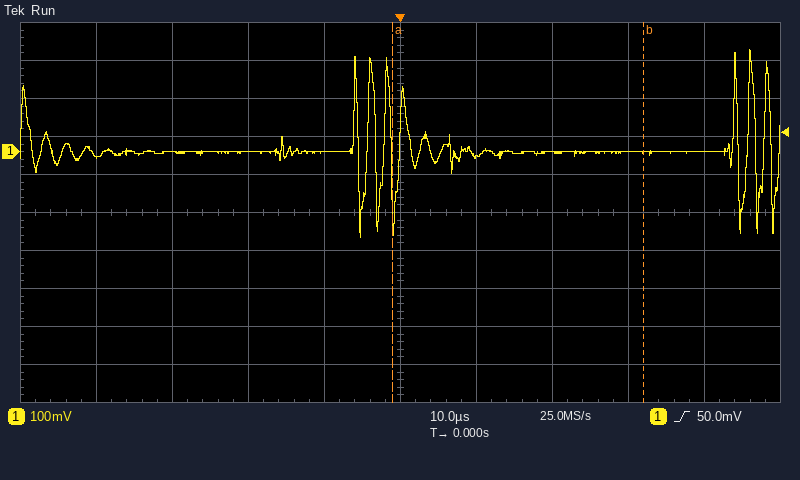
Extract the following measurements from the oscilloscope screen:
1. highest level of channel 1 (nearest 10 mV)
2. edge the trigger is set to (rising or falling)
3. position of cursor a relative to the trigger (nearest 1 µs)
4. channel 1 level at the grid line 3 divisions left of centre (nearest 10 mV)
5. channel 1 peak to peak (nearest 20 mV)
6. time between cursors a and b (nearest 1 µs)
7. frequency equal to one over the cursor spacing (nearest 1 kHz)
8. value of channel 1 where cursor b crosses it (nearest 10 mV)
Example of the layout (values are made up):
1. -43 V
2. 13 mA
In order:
1. 270 mV
2. rising
3. -1 µs
4. 0 mV
5. 500 mV
6. 33 µs
7. 30 kHz
8. 0 mV
